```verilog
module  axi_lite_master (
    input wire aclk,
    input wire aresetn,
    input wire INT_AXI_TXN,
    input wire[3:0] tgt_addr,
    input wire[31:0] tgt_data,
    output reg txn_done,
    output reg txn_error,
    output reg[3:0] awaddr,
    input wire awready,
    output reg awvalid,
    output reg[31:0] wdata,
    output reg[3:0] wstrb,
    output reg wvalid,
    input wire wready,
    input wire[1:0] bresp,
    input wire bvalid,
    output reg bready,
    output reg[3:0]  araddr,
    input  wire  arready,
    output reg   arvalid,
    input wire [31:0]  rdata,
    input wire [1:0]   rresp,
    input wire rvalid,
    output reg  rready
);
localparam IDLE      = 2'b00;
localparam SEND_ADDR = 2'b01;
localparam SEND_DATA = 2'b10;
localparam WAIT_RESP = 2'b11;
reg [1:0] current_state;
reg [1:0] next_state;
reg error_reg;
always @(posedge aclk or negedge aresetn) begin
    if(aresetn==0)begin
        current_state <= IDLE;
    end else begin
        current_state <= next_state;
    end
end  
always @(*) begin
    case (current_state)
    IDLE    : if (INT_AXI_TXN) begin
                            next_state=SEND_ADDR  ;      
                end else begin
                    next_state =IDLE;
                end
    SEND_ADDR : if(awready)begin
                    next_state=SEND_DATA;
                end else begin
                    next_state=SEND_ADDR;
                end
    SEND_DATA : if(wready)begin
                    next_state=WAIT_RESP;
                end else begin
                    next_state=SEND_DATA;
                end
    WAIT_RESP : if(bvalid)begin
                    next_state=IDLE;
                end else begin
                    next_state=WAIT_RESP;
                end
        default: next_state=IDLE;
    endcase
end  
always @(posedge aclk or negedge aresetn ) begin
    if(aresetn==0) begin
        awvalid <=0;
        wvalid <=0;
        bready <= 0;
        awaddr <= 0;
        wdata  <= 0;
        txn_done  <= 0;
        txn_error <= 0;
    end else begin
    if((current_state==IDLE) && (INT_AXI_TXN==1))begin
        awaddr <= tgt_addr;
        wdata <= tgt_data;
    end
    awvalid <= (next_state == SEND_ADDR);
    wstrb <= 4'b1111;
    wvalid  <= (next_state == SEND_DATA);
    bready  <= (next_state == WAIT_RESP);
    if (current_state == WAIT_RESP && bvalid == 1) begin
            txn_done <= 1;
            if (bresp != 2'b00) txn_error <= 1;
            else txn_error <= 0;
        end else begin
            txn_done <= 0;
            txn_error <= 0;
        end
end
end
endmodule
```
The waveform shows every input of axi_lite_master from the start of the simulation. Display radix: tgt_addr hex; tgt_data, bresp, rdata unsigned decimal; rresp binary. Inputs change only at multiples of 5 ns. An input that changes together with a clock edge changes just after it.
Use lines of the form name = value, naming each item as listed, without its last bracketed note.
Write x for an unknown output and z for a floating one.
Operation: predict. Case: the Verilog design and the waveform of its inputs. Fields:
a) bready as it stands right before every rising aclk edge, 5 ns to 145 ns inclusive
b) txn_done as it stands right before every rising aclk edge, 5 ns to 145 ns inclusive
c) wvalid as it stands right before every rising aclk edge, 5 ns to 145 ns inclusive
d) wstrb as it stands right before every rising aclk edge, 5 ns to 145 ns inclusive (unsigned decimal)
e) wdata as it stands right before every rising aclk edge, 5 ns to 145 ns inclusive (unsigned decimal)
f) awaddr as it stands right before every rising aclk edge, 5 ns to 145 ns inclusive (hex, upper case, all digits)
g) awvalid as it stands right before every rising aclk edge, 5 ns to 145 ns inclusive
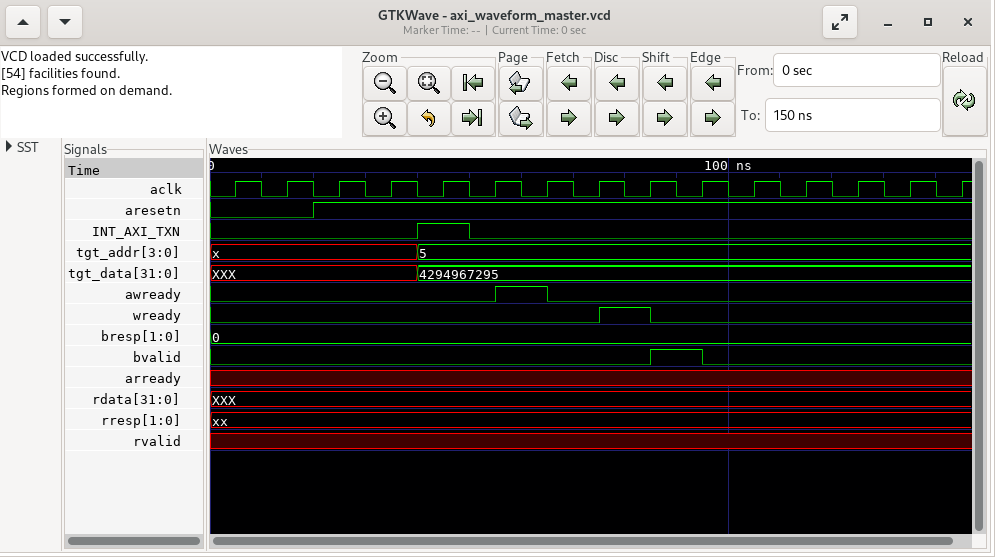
bready as it stands right before every rising aclk edge, 5 ns to 145 ns inclusive = 0 0 0 0 0 0 0 0 0 1 0 0 0 0 0
txn_done as it stands right before every rising aclk edge, 5 ns to 145 ns inclusive = 0 0 0 0 0 0 0 0 0 0 1 0 0 0 0
wvalid as it stands right before every rising aclk edge, 5 ns to 145 ns inclusive = 0 0 0 0 0 0 0 1 1 0 0 0 0 0 0
wstrb as it stands right before every rising aclk edge, 5 ns to 145 ns inclusive = x, x, x, 15, 15, 15, 15, 15, 15, 15, 15, 15, 15, 15, 15
wdata as it stands right before every rising aclk edge, 5 ns to 145 ns inclusive = 0, 0, 0, 0, 0, 4294967295, 4294967295, 4294967295, 4294967295, 4294967295, 4294967295, 4294967295, 4294967295, 4294967295, 4294967295
awaddr as it stands right before every rising aclk edge, 5 ns to 145 ns inclusive = 0, 0, 0, 0, 0, 5, 5, 5, 5, 5, 5, 5, 5, 5, 5
awvalid as it stands right before every rising aclk edge, 5 ns to 145 ns inclusive = 0 0 0 0 0 1 1 0 0 0 0 0 0 0 0
